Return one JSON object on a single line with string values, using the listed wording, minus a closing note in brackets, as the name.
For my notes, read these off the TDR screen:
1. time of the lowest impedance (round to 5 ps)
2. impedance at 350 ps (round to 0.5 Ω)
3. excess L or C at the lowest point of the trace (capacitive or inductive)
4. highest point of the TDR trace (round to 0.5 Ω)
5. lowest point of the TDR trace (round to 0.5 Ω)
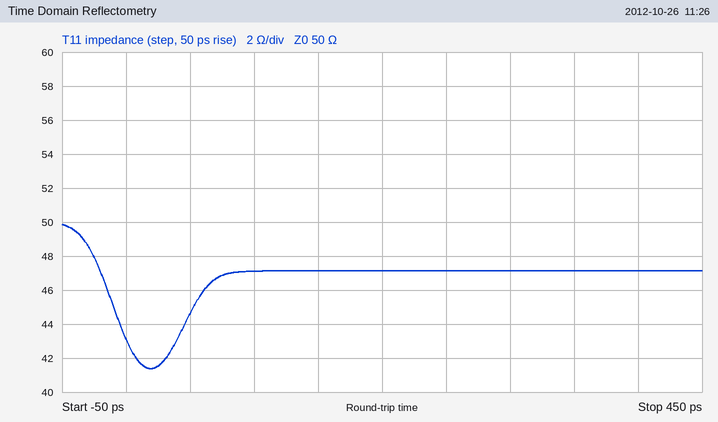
{"time of the lowest impedance": "20 ps", "impedance at 350 ps": "47.0 Ω", "excess L or C at the lowest point of the trace": "capacitive", "highest point of the TDR trace": "50.0 Ω", "lowest point of the TDR trace": "41.5 Ω"}
